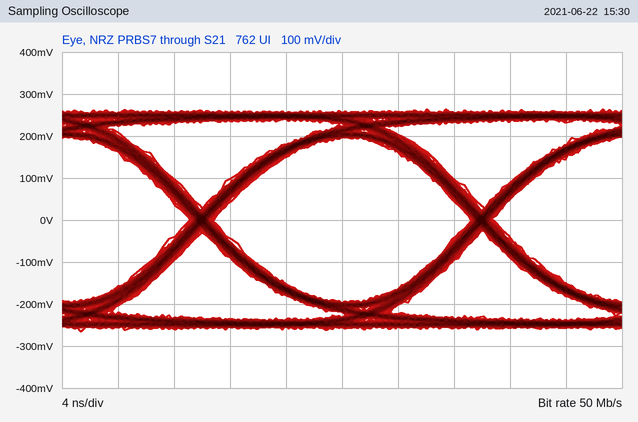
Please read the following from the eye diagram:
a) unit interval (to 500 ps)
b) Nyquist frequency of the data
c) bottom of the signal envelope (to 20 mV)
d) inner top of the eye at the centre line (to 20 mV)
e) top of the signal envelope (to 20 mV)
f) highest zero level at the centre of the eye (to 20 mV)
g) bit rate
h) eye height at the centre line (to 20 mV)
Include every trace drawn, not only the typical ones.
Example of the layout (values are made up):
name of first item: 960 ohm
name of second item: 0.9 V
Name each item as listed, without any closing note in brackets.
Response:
unit interval: 20.0 ns
Nyquist frequency of the data: 25 MHz
bottom of the signal envelope: -260 mV
inner top of the eye at the centre line: 200 mV
top of the signal envelope: 260 mV
highest zero level at the centre of the eye: -200 mV
bit rate: 50 Mb/s
eye height at the centre line: 400 mV
